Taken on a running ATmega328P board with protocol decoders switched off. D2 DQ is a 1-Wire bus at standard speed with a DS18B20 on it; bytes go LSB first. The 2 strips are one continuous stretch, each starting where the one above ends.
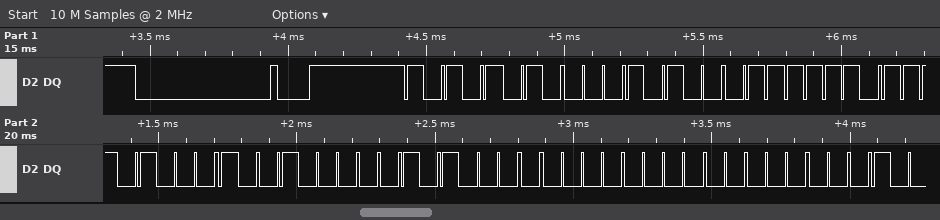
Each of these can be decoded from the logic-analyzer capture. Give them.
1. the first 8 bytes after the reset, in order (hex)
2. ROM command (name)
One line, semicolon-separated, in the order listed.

55 28 7E 17 09 0A 00 00; Match ROM
